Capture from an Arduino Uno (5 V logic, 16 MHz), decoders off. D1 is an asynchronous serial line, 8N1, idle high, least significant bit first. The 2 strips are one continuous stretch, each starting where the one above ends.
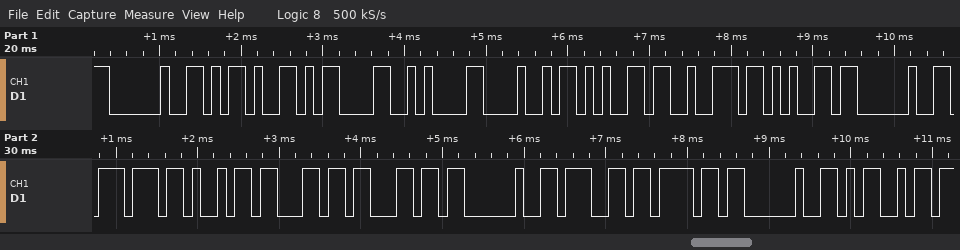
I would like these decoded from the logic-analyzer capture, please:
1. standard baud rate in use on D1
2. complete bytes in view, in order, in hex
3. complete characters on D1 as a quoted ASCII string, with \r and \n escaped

9600 baud
20 2D 0D 0A 48 65 72 65 20 77 69 6C 6C 20 67 6F 20 4D
" -\r\nHere will go M"
